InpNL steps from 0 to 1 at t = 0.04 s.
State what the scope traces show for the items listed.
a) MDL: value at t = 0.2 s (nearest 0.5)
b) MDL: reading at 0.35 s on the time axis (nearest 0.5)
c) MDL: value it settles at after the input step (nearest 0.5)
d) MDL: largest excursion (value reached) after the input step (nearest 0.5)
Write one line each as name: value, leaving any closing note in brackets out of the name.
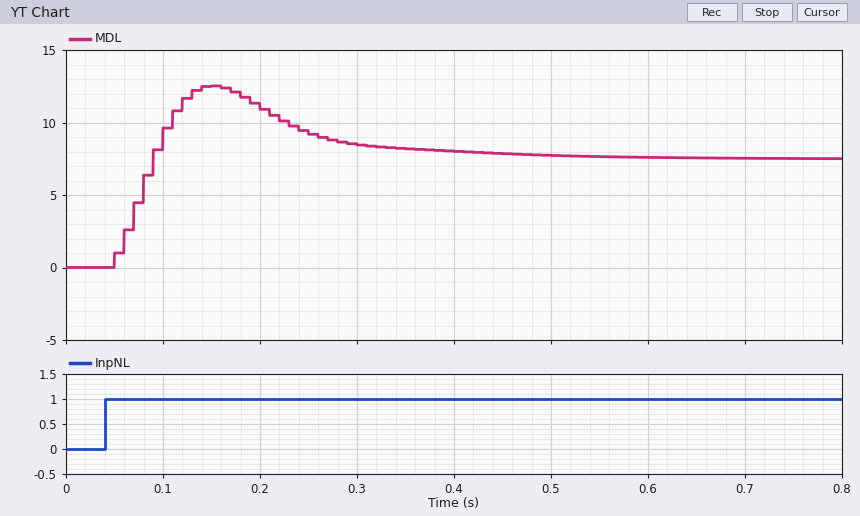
MDL: value at t = 0.2 s: 11.0
MDL: reading at 0.35 s on the time axis: 8.0
MDL: value it settles at after the input step: 7.5
MDL: largest excursion (value reached) after the input step: 12.5
